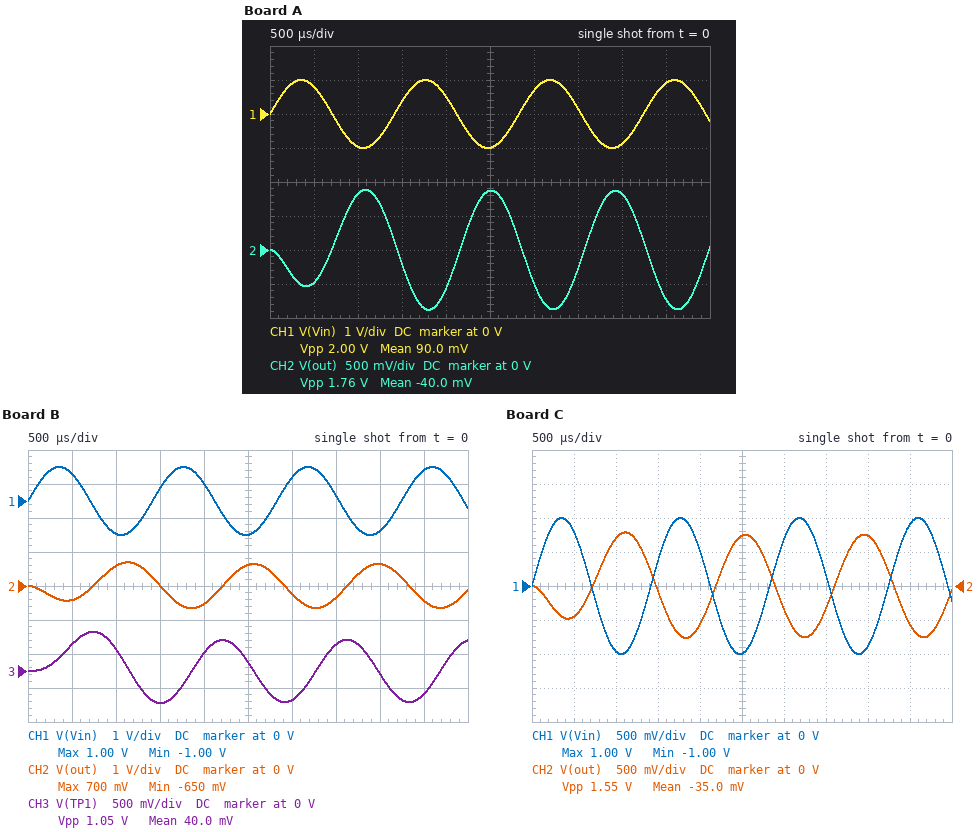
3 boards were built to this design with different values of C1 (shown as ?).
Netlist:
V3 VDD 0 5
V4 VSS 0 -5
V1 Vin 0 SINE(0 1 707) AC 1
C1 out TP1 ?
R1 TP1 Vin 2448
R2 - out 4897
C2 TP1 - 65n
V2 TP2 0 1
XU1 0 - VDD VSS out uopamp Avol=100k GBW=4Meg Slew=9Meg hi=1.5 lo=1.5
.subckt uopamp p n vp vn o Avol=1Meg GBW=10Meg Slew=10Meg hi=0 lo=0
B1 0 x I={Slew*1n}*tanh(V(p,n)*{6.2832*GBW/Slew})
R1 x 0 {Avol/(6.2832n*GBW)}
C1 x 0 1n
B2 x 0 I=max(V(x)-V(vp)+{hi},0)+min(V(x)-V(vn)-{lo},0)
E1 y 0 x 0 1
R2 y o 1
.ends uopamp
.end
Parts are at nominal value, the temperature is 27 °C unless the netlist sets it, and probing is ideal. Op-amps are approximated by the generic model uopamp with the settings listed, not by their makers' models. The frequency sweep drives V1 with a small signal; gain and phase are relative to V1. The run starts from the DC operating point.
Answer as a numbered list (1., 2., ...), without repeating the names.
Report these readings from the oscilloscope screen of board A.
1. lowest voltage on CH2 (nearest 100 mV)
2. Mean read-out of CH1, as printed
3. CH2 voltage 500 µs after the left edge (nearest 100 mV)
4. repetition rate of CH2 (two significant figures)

1. -900 mV
2. 90.0 mV
3. -500 mV
4. 700 Hz
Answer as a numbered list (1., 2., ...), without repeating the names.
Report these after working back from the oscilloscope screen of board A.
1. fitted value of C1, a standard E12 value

1. 82 nF
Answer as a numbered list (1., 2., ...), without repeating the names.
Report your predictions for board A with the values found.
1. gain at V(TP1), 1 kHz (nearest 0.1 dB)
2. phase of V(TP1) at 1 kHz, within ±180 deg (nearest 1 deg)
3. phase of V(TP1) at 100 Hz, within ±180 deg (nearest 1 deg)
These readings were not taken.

1. -8.7 dB
2. -124 deg
3. -13 deg
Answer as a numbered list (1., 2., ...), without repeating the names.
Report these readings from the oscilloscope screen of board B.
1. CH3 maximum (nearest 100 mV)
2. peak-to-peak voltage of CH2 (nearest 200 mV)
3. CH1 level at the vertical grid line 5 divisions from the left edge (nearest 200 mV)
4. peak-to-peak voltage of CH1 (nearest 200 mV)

1. 600 mV
2. 1.4 V
3. -1.0 V
4. 2.0 V
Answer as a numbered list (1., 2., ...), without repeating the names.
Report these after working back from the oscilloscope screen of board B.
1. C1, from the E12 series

1. 120 nF
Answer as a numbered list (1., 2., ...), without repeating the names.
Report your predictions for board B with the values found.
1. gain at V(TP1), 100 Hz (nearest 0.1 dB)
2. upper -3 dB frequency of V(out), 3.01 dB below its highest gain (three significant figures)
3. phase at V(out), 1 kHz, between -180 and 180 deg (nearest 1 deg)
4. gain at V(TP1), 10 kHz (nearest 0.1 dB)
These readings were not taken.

1. 0 dB
2. 1.03 kHz
3. 137 deg
4. -51.8 dB
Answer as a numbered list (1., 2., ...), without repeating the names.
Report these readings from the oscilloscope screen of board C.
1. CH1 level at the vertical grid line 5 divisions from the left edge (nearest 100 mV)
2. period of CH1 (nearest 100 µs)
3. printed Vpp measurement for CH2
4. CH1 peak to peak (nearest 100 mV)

1. -1.0 V
2. 1.4 ms
3. 1.55 V
4. 2.0 V
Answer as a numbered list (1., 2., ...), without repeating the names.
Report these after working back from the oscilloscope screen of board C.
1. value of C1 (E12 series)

1. 100 nF
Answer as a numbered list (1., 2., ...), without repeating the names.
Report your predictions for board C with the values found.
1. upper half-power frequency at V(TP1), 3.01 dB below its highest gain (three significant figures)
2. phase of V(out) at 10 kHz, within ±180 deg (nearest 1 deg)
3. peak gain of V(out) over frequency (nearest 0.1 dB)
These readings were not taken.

1. 557 Hz
2. 95 deg
3. -2.1 dB
